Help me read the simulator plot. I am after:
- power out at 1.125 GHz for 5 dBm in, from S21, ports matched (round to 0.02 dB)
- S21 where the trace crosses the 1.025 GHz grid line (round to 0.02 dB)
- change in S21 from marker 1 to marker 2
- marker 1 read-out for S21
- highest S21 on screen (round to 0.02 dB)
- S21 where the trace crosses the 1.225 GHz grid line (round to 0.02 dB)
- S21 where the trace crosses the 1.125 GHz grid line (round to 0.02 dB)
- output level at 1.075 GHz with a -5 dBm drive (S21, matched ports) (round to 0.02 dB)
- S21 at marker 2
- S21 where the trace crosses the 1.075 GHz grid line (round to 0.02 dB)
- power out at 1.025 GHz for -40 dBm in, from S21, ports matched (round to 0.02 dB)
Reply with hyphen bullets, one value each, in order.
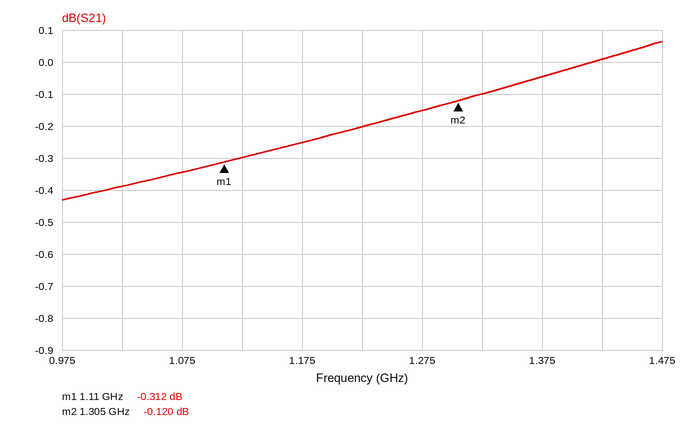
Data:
- 4.70 dBm
- -0.38 dB
- 0.192 dB
- -0.312 dB
- 0.06 dB
- -0.20 dB
- -0.30 dB
- -5.34 dBm
- -0.120 dB
- -0.34 dB
- -40.38 dBm
